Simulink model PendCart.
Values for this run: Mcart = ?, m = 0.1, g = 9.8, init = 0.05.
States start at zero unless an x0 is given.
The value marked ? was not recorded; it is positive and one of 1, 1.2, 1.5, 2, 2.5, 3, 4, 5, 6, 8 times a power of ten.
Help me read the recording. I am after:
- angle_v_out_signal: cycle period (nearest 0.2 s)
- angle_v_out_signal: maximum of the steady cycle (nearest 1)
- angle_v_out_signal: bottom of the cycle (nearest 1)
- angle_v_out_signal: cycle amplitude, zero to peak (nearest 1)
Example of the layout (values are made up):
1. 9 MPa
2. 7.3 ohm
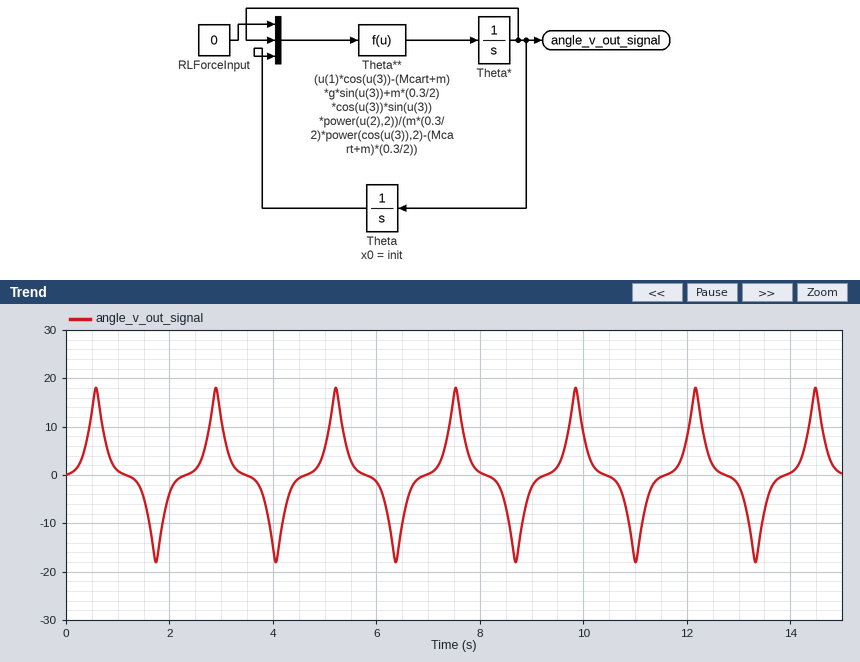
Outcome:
1. 2.4 s
2. 18
3. -18
4. 18
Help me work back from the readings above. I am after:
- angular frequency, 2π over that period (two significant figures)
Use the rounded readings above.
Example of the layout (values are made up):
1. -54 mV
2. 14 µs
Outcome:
1. 2.6 rad/s
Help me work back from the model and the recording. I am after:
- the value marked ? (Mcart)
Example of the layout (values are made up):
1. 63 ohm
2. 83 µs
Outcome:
1. 0.4
